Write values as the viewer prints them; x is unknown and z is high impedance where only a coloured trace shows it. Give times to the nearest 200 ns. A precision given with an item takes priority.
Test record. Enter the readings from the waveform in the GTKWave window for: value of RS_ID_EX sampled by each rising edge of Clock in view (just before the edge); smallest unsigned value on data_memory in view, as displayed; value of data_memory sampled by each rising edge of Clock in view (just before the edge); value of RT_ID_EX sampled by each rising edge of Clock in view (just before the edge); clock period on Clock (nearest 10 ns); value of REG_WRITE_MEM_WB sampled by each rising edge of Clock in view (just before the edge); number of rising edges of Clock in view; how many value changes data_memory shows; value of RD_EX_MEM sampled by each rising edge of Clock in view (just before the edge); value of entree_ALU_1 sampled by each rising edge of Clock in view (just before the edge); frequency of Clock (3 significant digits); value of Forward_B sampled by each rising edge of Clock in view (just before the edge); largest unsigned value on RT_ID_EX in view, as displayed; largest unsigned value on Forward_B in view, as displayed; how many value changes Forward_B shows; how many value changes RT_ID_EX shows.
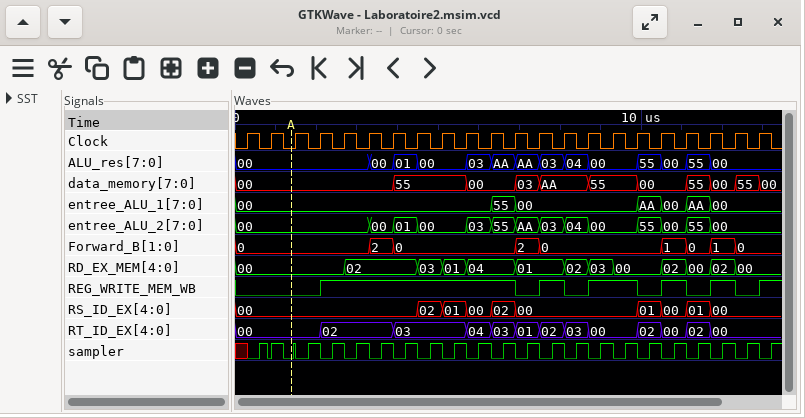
00, 00, 00, 00, 00, 00, 00, 00, 02, 01, 00, 02, 00, 00, 00, 00, 00, 01, 00, 01, 00, 00
00
00, 00, 00, 00, 00, 00, 00, 55, 55, 55, 00, 00, 03, AA, AA, 55, 55, 00, 00, 55, 00, 55
00, 00, 00, 00, 02, 02, 02, 03, 03, 03, 04, 03, 01, 02, 03, 00, 00, 02, 00, 02, 00, 00
600 ns
0 0 0 0 1 1 1 1 1 1 1 1 0 1 0 1 1 0 1 0 1 0
22
10
00, 00, 00, 00, 00, 02, 02, 02, 03, 01, 04, 04, 01, 01, 02, 03, 00, 00, 02, 00, 02, 00
00, 00, 00, 00, 00, 00, 00, 00, 00, 00, 00, 55, 00, 00, 00, 00, 00, AA, 00, AA, 00, 00
1.67 MHz
0, 0, 0, 0, 0, 0, 2, 0, 0, 0, 0, 0, 2, 0, 0, 0, 0, 0, 1, 0, 1, 0
04
2
8
12
